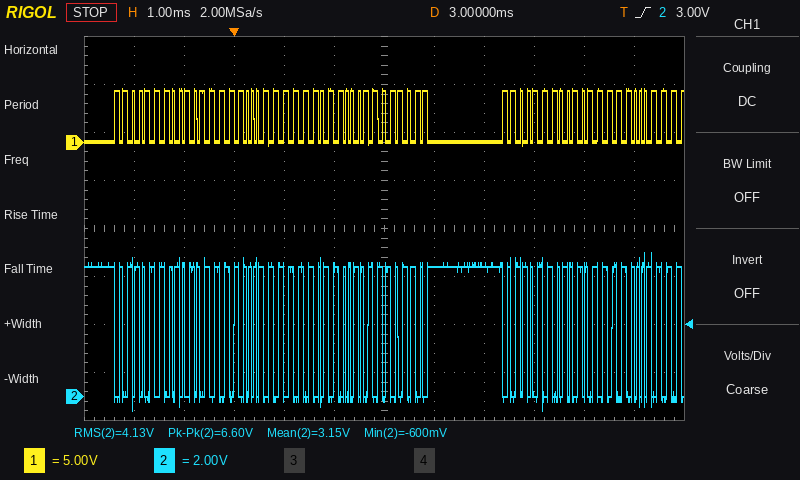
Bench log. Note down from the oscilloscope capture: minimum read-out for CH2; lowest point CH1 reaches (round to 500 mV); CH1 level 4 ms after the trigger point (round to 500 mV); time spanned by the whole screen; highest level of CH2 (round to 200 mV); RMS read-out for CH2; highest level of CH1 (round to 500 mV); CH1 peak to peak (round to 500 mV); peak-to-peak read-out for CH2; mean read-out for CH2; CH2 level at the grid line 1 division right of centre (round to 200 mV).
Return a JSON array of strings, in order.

["-600 mV", "-500 mV", "0.0 V", "12 ms", "6.0 V", "4.13 V", "5.5 V", "6.0 V", "6.60 V", "3.15 V", "5.4 V"]
